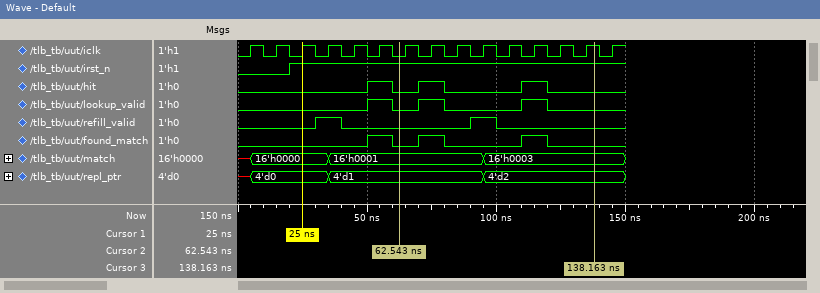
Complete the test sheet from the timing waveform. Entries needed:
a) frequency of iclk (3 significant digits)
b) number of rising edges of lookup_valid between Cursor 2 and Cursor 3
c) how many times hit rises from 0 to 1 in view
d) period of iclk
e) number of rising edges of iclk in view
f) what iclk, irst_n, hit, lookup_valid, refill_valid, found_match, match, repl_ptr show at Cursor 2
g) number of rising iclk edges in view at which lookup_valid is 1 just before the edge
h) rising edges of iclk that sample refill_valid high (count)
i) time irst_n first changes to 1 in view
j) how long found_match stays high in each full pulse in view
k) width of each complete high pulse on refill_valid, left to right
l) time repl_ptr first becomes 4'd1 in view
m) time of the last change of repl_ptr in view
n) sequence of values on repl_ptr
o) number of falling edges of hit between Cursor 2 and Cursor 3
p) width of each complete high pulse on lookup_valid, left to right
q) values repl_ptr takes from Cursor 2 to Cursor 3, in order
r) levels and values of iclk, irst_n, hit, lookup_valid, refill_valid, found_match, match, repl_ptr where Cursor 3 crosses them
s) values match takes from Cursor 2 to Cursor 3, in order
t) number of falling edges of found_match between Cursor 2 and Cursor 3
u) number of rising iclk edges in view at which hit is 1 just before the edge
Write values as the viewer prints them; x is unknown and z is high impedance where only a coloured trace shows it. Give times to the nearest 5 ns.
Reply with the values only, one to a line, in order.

100 MHz
2
3
10 ns
15
iclk=0, irst_n=1, hit=0, lookup_valid=0, refill_valid=0, found_match=0, match=16'h0001, repl_ptr=4'd1
3
2
20 ns
10 ns, 10 ns, 10 ns
10 ns, 10 ns
35 ns
95 ns
x, 4'd0, 4'd1, 4'd2
2
10 ns, 10 ns, 10 ns
4'd1, 4'd2
iclk=1, irst_n=1, hit=0, lookup_valid=0, refill_valid=0, found_match=0, match=16'h0003, repl_ptr=4'd2
16'h0001, 16'h0003
2
3
